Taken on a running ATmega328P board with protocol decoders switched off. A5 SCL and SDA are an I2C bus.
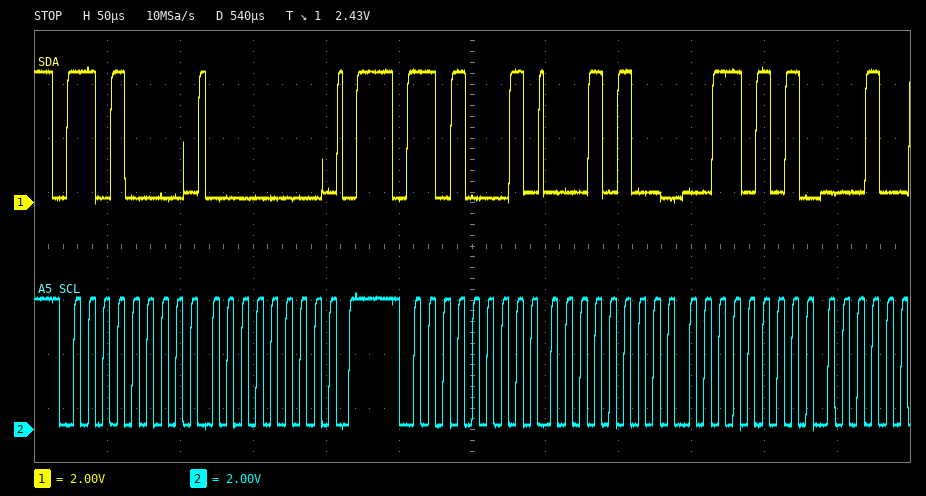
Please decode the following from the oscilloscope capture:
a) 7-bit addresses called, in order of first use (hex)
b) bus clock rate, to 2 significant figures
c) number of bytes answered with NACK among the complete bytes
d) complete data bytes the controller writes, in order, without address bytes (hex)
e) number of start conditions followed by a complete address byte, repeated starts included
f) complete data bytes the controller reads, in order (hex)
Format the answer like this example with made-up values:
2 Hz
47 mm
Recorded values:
0x68
100 kHz
0
00
2
14 35
